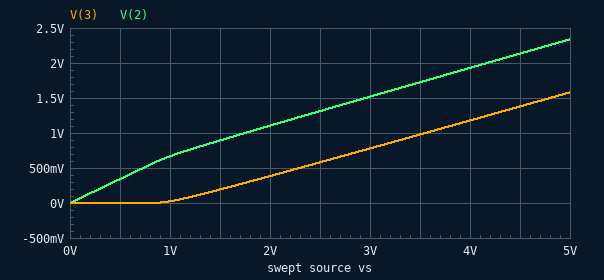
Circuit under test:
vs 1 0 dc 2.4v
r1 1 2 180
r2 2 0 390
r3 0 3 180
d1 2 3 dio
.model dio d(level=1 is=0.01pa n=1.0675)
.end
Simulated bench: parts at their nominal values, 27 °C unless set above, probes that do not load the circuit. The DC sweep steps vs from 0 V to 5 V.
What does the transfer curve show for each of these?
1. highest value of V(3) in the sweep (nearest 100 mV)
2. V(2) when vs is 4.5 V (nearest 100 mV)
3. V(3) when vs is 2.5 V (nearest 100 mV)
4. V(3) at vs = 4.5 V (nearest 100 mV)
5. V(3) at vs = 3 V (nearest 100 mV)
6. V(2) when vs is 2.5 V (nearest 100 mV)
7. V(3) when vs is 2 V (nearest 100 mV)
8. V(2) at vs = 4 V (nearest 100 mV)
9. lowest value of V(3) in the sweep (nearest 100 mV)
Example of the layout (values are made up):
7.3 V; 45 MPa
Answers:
1.6 V; 2.1 V; 600 mV; 1.4 V; 800 mV; 1.3 V; 400 mV; 1.9 V; 0 V
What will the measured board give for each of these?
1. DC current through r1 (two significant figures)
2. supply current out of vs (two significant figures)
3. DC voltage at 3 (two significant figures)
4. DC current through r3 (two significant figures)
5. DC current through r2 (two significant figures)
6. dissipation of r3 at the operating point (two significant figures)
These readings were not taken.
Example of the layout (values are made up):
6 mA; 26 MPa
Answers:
6.3 mA; 6.3 mA; 540 mV; 3.0 mA; 3.3 mA; 1.6 mW
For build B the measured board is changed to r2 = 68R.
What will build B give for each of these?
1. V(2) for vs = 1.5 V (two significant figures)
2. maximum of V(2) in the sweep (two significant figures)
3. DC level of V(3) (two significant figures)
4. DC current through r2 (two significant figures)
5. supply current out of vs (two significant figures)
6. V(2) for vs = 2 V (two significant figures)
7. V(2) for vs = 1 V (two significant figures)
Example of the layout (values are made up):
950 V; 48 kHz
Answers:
410 mV; 1.2 V; 18 mV; 9.6 mA; 9.7 mA; 550 mV; 270 mV
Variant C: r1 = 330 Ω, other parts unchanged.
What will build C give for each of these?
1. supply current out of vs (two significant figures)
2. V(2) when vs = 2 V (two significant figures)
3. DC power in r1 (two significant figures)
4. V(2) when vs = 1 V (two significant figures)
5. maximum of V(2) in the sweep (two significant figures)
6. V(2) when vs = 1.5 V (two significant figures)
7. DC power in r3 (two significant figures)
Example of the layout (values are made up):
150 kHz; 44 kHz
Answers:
4.2 mA; 890 mV; 5.9 mW; 540 mV; 1.7 V; 740 mV; 480 µW
